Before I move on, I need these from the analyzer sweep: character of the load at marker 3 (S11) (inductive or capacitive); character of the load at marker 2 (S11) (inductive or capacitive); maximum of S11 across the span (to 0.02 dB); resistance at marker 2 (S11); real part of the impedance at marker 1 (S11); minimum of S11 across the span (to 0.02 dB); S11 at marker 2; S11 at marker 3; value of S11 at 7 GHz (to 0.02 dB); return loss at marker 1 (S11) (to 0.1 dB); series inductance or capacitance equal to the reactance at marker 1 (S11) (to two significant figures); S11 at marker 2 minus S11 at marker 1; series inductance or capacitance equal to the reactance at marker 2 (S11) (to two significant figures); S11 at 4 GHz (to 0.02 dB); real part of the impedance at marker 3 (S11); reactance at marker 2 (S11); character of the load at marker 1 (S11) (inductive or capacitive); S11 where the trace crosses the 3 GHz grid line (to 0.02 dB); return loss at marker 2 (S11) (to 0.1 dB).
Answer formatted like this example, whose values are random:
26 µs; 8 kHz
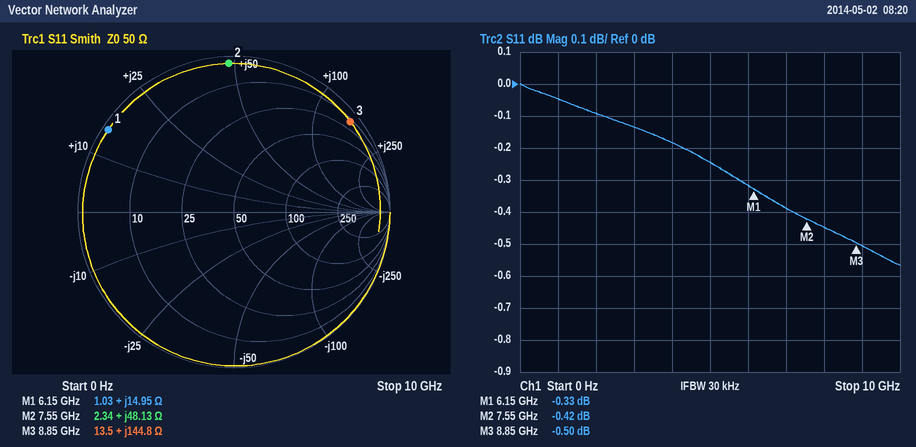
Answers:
inductive; inductive; 0.00 dB; 2.34 Ω; 1.03 Ω; -0.56 dB; -0.42 dB; -0.50 dB; -0.38 dB; 0.3 dB; 390 pH; -0.09 dB; 1.0 nH; -0.18 dB; 13.5 Ω; +48.13 Ω; inductive; -0.14 dB; 0.4 dB
